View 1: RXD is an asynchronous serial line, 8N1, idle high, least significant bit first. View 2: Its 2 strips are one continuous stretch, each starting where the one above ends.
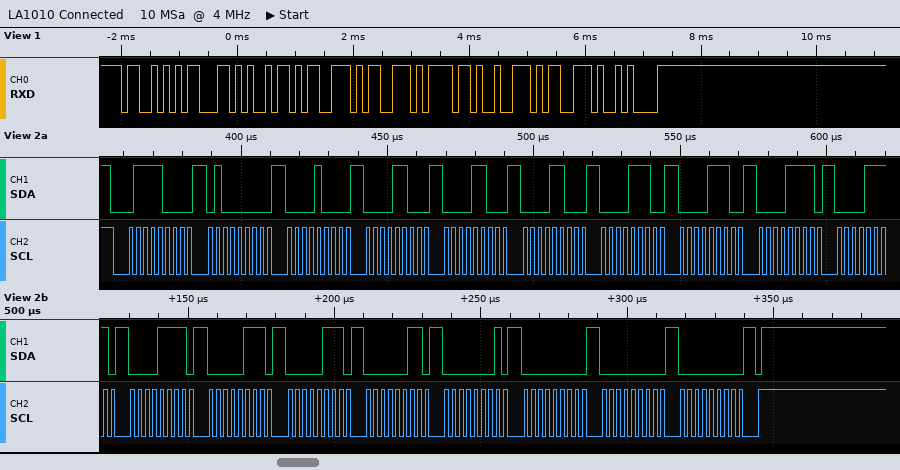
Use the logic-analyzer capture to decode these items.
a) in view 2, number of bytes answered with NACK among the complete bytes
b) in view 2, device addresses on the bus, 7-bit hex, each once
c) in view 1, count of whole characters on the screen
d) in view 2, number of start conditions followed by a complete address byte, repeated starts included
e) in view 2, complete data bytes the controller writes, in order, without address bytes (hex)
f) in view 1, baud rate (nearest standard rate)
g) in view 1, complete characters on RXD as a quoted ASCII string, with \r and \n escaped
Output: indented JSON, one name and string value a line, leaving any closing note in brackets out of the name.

{
  "in view 2, number of bytes answered with NACK among the complete bytes": "0",
  "in view 2, device addresses on the bus, 7-bit hex, each once": "0x3C",
  "in view 1, count of whole characters on the screen": "9",
  "in view 2, number of start conditions followed by a complete address byte, repeated starts included": "1",
  "in view 2, complete data bytes the controller writes, in order, without address bytes": "40 08 0C 0C 0C 0E 0E 0F 0F 0F 07 07 03 01 00 00 00",
  "in view 1, baud rate": "9600 baud",
  "in view 1, complete characters on RXD as a quoted ASCII string, with \\r and \\n escaped": "\"Scissors\\n\""
}
